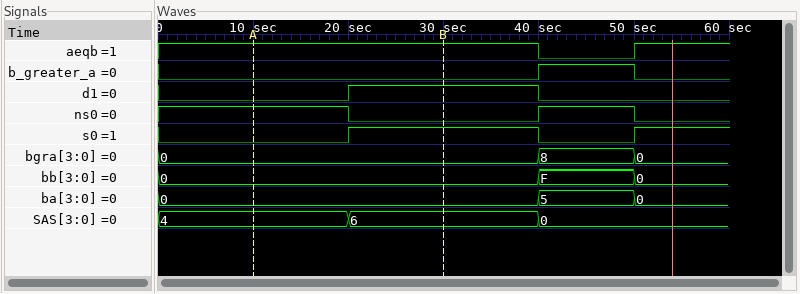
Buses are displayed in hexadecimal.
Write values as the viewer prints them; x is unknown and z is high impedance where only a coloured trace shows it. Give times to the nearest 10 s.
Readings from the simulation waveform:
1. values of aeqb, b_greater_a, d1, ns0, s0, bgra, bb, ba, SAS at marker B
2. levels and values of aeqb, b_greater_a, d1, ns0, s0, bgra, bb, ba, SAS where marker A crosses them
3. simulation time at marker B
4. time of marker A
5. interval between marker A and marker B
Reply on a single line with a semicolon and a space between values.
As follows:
aeqb=1, b_greater_a=0, d1=1, ns0=0, s0=1, bgra=0, bb=0, ba=0, SAS=6; aeqb=1, b_greater_a=0, d1=0, ns0=1, s0=0, bgra=0, bb=0, ba=0, SAS=4; 30 s; 10 s; 20 s
